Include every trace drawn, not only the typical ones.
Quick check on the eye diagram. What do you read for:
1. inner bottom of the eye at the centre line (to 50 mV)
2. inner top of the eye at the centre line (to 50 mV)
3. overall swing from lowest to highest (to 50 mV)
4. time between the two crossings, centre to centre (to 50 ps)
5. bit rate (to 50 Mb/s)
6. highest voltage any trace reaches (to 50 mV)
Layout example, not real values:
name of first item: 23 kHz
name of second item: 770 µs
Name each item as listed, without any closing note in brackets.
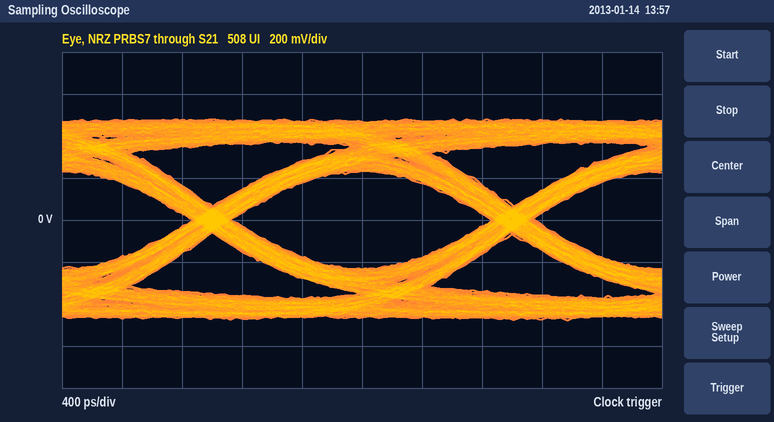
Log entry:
inner bottom of the eye at the centre line: -250 mV
inner top of the eye at the centre line: 250 mV
overall swing from lowest to highest: 950 mV
time between the two crossings, centre to centre: 2.00 ns
bit rate: 500 Mb/s
highest voltage any trace reaches: 500 mV
